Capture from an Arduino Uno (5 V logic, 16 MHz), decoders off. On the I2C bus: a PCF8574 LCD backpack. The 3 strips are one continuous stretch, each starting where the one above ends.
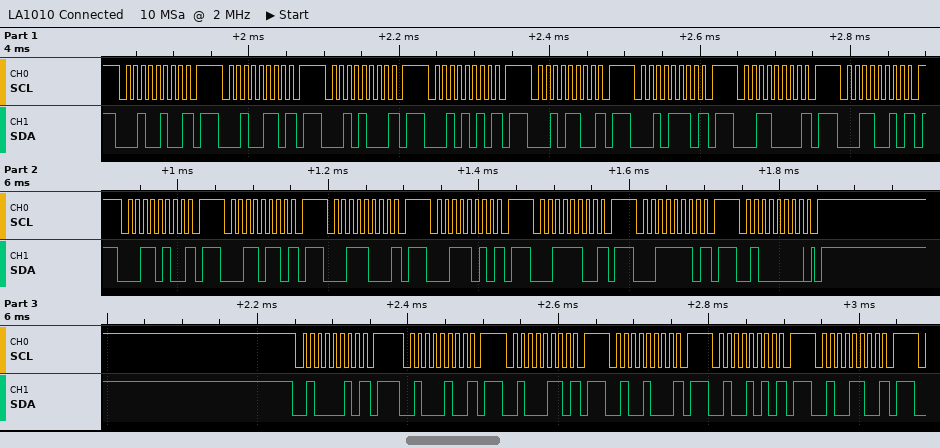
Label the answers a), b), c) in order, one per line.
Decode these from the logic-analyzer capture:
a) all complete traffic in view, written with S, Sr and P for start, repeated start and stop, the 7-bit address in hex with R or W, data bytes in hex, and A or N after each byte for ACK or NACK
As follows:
a) S 12W N P S 13W N P S 14W N P S 15W N P S 16W N P S 17W N P S 18W N P S 19W N P S 1AW N P S 1BW N P S 1CW N P S 1DW N P S 1EW N P S 1FW N P S 20W A P S 21W N P S 22W N P S 23W N P S 24W N P S 25W N P S 26W N P
